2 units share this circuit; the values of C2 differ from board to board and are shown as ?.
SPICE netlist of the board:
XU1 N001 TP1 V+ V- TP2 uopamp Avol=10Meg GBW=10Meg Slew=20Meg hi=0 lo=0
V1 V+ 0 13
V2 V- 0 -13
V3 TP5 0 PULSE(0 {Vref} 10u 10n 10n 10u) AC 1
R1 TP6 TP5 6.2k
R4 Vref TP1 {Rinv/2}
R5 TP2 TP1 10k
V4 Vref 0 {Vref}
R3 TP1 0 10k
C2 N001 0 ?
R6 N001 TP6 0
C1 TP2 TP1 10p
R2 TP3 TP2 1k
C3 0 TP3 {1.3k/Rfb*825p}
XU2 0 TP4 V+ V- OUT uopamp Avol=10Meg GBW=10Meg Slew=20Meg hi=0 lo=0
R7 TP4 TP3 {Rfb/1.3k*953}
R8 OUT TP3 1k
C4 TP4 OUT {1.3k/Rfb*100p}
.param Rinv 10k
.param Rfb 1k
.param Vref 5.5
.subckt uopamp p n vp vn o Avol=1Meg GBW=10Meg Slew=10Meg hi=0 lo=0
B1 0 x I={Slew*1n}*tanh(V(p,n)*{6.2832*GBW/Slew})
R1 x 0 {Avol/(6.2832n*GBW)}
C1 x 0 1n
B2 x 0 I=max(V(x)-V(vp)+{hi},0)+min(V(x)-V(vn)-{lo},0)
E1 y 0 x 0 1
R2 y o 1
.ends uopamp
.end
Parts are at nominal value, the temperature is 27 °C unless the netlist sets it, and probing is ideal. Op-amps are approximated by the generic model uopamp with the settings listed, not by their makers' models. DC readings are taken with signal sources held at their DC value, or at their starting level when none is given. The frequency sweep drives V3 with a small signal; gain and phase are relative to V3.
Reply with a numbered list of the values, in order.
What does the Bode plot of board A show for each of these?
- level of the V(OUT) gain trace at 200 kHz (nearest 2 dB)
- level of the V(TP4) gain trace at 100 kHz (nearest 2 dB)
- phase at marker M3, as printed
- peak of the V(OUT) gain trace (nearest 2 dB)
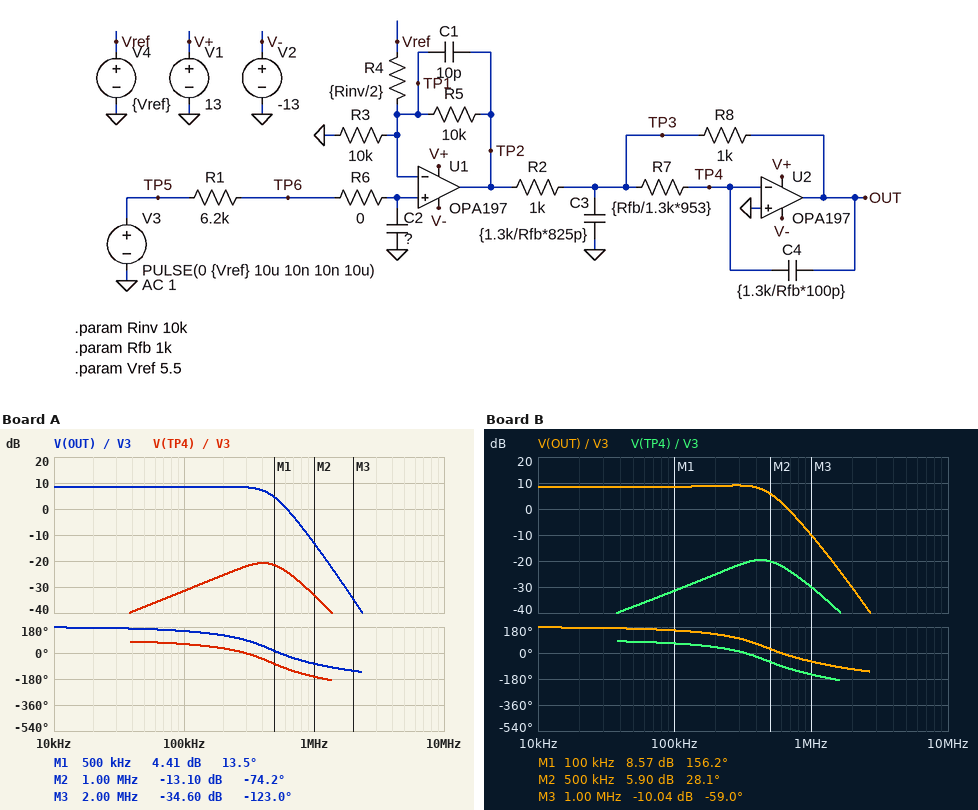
1. 8 dB
2. -32 dB
3. -123.0 deg
4. 8 dB
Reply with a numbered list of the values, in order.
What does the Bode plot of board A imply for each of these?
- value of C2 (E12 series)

1. 68 pF
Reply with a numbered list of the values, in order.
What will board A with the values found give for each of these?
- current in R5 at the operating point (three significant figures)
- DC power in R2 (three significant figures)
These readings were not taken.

1. 1.10 mA
2. 121 mW
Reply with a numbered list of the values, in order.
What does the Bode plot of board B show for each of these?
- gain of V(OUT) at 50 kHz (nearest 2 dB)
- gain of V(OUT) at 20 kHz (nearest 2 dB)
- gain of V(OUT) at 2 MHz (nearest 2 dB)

1. 8 dB
2. 8 dB
3. -30 dB
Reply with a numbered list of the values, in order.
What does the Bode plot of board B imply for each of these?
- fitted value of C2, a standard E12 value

1. 39 pF
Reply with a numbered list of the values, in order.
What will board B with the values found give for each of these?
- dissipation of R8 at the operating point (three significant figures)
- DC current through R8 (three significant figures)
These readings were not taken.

1. 121 mW
2. 11.0 mA
